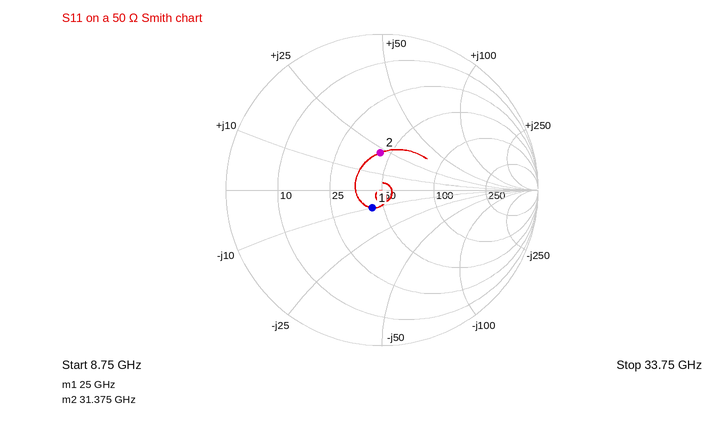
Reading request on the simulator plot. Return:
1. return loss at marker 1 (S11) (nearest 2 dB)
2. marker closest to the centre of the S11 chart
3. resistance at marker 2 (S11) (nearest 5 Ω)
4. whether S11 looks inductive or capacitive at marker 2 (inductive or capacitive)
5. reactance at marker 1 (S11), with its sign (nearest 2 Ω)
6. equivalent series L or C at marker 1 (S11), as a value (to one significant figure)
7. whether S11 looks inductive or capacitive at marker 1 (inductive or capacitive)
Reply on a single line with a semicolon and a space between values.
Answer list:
18 dB; marker 1; 45 Ω; inductive; -10 Ω; 600 fF; capacitive
